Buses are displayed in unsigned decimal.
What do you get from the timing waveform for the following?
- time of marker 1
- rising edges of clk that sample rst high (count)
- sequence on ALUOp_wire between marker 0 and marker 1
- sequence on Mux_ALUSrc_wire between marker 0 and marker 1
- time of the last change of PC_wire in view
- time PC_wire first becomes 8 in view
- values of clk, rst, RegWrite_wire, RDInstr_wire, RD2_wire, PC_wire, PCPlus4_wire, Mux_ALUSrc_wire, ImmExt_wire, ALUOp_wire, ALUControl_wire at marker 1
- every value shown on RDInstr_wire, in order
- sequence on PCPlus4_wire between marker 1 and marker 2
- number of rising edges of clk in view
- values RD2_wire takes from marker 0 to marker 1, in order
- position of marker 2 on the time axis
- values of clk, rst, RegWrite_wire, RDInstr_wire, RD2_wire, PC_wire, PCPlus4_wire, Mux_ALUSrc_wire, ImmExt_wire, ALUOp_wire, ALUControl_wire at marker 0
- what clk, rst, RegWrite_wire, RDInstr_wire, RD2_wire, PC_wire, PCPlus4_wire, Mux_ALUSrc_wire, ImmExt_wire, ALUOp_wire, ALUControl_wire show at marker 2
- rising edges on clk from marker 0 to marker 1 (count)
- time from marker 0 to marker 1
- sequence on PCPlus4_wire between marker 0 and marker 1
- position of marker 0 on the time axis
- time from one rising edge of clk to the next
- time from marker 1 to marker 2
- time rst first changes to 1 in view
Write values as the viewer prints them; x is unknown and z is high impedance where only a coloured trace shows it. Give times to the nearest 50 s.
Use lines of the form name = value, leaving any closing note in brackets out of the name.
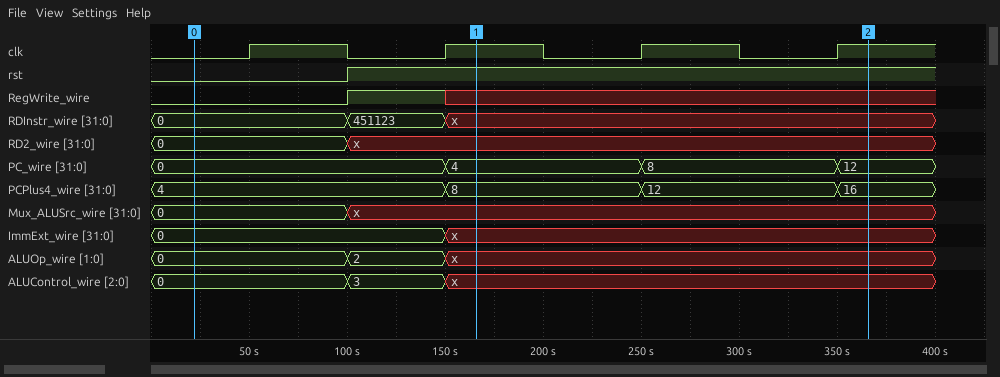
time of marker 1 = 150 s
rising edges of clk that sample rst high = 3
sequence on ALUOp_wire between marker 0 and marker 1 = 0, 2, x
sequence on Mux_ALUSrc_wire between marker 0 and marker 1 = 0, x
time of the last change of PC_wire in view = 350 s
time PC_wire first becomes 8 in view = 250 s
values of clk, rst, RegWrite_wire, RDInstr_wire, RD2_wire, PC_wire, PCPlus4_wire, Mux_ALUSrc_wire, ImmExt_wire, ALUOp_wire, ALUControl_wire at marker 1 = clk=1, rst=1, RegWrite_wire=x, RDInstr_wire=x, RD2_wire=x, PC_wire=4, PCPlus4_wire=8, Mux_ALUSrc_wire=x, ImmExt_wire=x, ALUOp_wire=x, ALUControl_wire=x
every value shown on RDInstr_wire, in order = 0, 451123, x
sequence on PCPlus4_wire between marker 1 and marker 2 = 8, 12, 16
number of rising edges of clk in view = 4
values RD2_wire takes from marker 0 to marker 1, in order = 0, x
position of marker 2 on the time axis = 350 s
values of clk, rst, RegWrite_wire, RDInstr_wire, RD2_wire, PC_wire, PCPlus4_wire, Mux_ALUSrc_wire, ImmExt_wire, ALUOp_wire, ALUControl_wire at marker 0 = clk=0, rst=0, RegWrite_wire=0, RDInstr_wire=0, RD2_wire=0, PC_wire=0, PCPlus4_wire=4, Mux_ALUSrc_wire=0, ImmExt_wire=0, ALUOp_wire=0, ALUControl_wire=0
what clk, rst, RegWrite_wire, RDInstr_wire, RD2_wire, PC_wire, PCPlus4_wire, Mux_ALUSrc_wire, ImmExt_wire, ALUOp_wire, ALUControl_wire show at marker 2 = clk=1, rst=1, RegWrite_wire=x, RDInstr_wire=x, RD2_wire=x, PC_wire=12, PCPlus4_wire=16, Mux_ALUSrc_wire=x, ImmExt_wire=x, ALUOp_wire=x, ALUControl_wire=x
rising edges on clk from marker 0 to marker 1 = 2
time from marker 0 to marker 1 = 150 s
sequence on PCPlus4_wire between marker 0 and marker 1 = 4, 8
position of marker 0 on the time axis = 0 s
time from one rising edge of clk to the next = 100 s
time from marker 1 to marker 2 = 200 s
time rst first changes to 1 in view = 100 s
